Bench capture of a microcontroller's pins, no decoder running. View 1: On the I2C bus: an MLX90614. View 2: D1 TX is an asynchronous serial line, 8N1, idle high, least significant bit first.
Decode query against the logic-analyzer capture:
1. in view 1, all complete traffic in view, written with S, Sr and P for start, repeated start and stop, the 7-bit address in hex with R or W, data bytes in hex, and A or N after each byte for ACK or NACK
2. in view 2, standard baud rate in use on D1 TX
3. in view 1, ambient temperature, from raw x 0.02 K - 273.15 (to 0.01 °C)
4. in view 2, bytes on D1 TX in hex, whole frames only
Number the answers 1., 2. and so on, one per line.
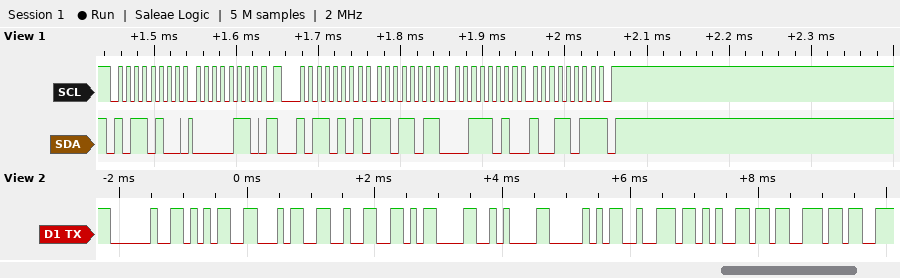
1. S 5AW A 06 A Sr 5AR A DB A 3A A 9B N P
2. 9600 baud
3. 28.19 °C
4. 20 35 34 32 0D 0A 50 72 65 73
